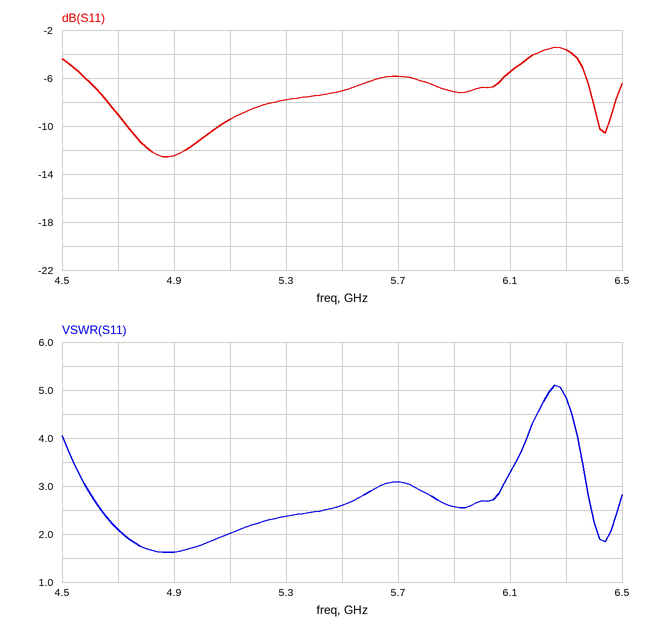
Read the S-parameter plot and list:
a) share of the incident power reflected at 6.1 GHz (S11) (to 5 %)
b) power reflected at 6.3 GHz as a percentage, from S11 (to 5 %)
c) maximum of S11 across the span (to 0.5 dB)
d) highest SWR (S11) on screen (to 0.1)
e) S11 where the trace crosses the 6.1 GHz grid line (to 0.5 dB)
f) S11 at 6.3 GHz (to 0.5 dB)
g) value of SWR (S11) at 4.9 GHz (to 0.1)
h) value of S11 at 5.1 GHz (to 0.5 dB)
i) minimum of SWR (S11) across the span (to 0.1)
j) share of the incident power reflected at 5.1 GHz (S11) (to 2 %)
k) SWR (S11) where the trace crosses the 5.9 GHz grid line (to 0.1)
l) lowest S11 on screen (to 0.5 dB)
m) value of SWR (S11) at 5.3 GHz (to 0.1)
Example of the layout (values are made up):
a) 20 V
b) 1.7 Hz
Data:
a) 30 %
b) 45 %
c) -3.5 dB
d) 5.1
e) -5.5 dB
f) -3.5 dB
g) 1.6
h) -9.5 dB
i) 1.6
j) 12 %
k) 2.6
l) -12.5 dB
m) 2.4
